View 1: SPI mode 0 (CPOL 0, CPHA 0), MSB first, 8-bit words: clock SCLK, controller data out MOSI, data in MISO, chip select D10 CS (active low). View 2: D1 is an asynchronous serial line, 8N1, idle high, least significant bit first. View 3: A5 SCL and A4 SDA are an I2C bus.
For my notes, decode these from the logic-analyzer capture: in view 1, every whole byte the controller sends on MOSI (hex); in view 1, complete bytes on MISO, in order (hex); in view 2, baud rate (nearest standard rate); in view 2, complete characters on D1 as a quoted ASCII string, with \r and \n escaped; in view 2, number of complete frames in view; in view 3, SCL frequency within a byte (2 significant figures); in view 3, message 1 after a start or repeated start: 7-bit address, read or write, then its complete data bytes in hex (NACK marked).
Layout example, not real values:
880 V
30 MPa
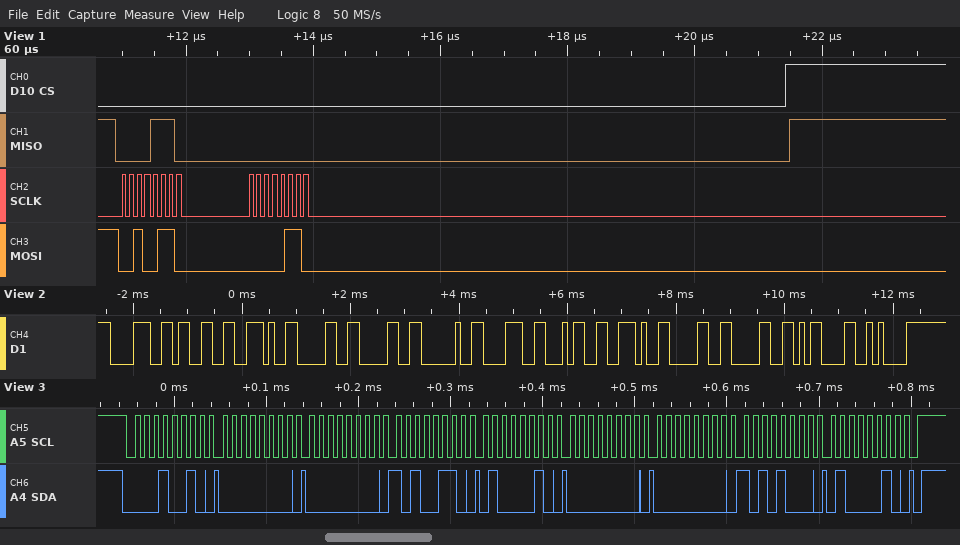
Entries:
0x26 0x06
0x0E 0x00
9600 baud
"83.00 84.00\r\n"
13
100 kHz
0x09 write: 00 00 A6 42 00 00 A8 42
